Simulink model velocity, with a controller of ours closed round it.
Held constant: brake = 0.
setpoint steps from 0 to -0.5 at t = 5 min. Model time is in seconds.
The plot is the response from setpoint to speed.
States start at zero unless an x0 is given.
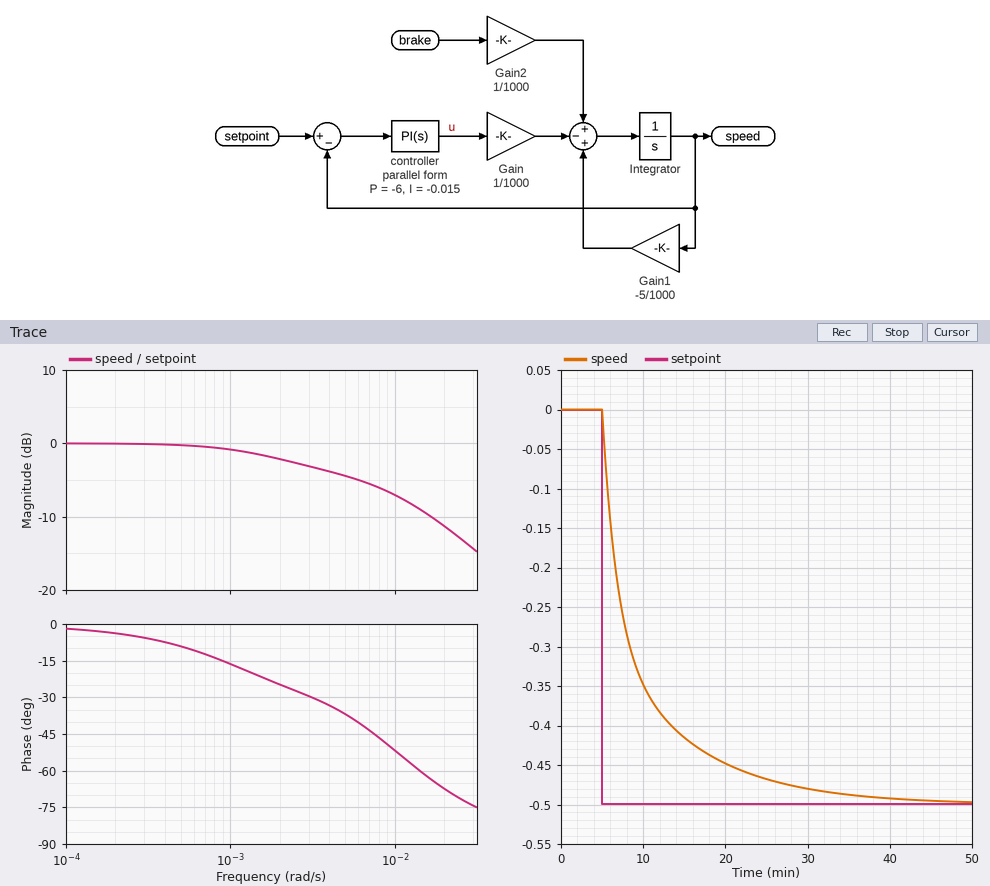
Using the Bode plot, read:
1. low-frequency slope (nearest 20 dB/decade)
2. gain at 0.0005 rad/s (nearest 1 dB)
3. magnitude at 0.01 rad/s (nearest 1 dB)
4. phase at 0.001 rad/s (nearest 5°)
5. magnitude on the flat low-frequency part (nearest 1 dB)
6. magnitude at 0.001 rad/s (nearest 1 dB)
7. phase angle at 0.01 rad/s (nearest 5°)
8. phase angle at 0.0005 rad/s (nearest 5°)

0 dB/decade
0 dB
-7 dB
-15°
0 dB
-1 dB
-50°
-10°
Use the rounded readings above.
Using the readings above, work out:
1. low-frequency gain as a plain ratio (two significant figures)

1.0
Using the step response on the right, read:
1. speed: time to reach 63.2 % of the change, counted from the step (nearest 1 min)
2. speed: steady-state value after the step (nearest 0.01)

4 min
-0.50
